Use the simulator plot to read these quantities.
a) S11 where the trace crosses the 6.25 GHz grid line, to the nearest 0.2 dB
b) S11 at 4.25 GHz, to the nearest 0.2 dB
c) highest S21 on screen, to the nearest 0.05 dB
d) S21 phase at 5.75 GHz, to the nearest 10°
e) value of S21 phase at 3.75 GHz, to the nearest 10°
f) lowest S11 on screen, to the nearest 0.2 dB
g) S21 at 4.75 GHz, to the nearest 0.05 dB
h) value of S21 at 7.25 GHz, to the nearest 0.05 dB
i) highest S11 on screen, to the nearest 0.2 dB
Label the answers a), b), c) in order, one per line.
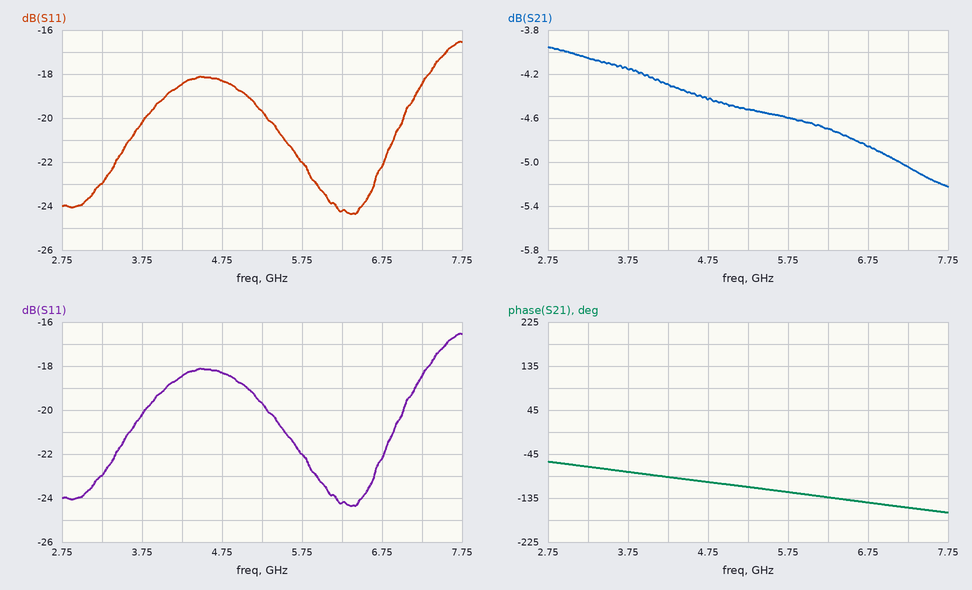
a) -24.2 dB
b) -18.4 dB
c) -3.95 dB
d) -120°
e) -80°
f) -24.4 dB
g) -4.45 dB
h) -5.05 dB
i) -16.6 dB
